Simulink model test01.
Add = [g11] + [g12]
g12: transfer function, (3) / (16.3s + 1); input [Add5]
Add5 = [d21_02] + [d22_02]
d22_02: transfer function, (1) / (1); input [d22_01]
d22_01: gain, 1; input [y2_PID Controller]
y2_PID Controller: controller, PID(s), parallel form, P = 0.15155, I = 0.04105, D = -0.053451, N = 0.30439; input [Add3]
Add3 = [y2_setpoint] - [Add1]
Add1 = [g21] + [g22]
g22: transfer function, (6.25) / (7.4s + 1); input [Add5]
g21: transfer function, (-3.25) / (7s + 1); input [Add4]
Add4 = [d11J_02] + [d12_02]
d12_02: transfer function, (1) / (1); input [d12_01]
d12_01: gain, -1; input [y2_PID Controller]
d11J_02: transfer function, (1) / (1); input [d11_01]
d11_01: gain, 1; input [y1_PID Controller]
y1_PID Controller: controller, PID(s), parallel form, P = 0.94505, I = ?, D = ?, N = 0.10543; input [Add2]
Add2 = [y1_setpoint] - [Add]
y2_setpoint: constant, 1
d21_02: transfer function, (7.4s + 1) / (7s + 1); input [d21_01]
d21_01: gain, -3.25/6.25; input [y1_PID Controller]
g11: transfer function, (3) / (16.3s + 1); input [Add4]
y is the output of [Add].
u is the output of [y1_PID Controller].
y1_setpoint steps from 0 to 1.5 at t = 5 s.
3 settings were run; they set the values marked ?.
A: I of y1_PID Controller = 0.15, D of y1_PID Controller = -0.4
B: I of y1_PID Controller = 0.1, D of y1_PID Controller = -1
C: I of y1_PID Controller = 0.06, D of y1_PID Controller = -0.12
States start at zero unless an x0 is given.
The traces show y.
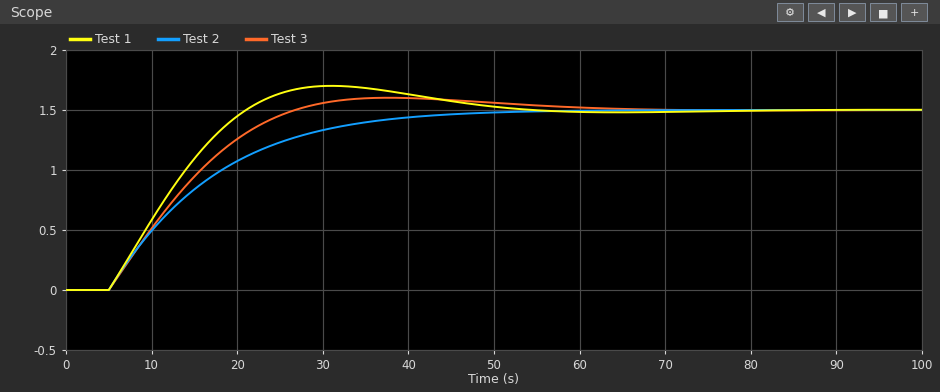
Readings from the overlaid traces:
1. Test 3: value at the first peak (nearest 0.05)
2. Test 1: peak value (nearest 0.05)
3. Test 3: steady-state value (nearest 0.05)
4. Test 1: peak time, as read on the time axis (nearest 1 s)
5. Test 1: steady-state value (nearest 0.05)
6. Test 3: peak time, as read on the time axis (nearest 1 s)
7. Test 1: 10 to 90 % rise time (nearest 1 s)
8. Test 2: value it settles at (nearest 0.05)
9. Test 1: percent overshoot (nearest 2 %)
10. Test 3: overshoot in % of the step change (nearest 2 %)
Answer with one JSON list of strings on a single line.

["1.60", "1.70", "1.50", "31 s", "1.50", "38 s", "12 s", "1.50", "14 %", "6 %"]
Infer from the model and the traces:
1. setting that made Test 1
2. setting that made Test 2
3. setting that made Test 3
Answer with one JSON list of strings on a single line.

["A", "C", "B"]
